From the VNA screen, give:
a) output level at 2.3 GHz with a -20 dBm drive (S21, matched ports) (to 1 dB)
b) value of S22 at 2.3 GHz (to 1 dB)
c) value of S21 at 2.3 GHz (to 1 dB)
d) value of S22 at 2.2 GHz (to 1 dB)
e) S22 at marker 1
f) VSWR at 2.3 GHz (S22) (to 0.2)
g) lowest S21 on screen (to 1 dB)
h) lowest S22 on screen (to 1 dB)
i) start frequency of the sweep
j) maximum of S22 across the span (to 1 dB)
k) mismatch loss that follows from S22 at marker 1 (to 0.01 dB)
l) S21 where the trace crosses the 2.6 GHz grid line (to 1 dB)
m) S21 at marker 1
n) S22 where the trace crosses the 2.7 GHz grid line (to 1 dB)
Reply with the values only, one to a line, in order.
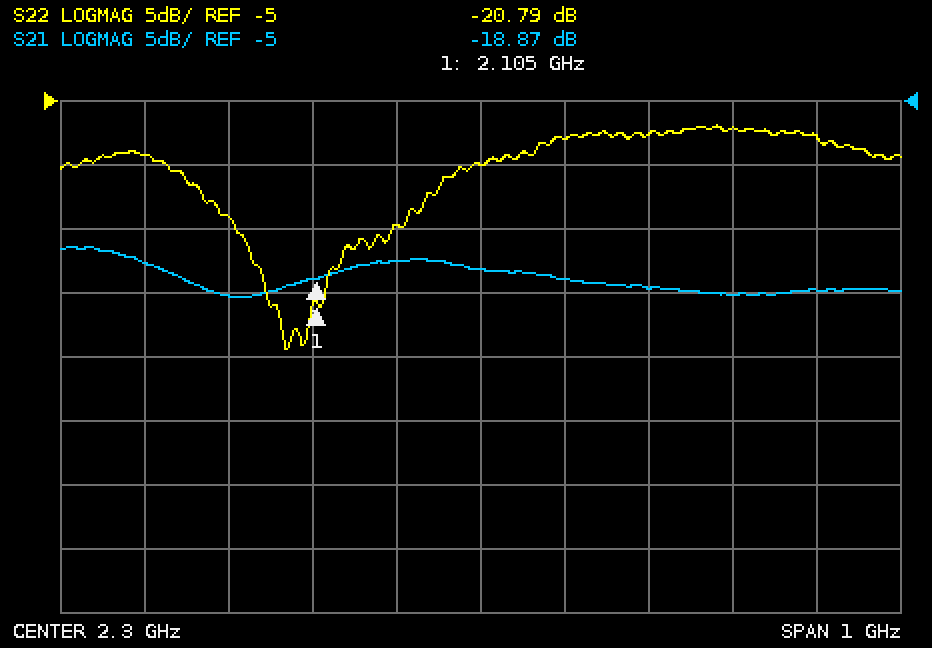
-38 dBm
-10 dB
-18 dB
-15 dB
-20.79 dB
2.0
-20 dB
-24 dB
1.8 GHz
-7 dB
0.04 dB
-20 dB
-18.87 dB
-8 dB
